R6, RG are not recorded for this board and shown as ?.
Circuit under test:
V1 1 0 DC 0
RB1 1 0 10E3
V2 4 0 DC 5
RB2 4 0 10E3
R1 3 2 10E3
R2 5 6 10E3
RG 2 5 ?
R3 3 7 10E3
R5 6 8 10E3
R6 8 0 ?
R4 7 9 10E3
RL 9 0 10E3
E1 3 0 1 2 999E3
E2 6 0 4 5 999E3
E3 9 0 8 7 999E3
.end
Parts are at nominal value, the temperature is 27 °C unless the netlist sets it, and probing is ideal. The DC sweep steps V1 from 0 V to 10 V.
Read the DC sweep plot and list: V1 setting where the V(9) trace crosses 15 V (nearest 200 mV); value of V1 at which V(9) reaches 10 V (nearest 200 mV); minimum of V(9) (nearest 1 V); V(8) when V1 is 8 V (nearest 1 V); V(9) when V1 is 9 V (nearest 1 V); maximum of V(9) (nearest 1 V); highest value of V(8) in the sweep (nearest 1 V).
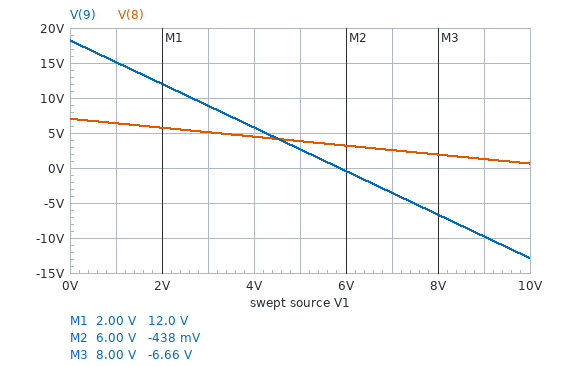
1.0 V
2.6 V
-13 V
2 V
-10 V
18 V
7 V
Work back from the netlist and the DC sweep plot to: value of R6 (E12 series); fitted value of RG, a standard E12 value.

33 kΩ
12 kΩ
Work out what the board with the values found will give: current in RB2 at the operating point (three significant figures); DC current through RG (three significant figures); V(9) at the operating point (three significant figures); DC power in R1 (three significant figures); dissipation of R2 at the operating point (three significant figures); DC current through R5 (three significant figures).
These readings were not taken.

500 µA
417 µA
18.2 V
1.74 mW
1.74 mW
213 µA
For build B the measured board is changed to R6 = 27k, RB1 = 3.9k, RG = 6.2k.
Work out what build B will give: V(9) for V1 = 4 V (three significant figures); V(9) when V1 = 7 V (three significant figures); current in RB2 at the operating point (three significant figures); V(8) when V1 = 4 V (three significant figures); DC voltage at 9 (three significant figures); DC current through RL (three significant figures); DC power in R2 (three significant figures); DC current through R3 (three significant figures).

7.26 V
-7.64 V
500 µA
4.83 V
27.1 V
2.71 mA
6.50 mW
1.76 mA
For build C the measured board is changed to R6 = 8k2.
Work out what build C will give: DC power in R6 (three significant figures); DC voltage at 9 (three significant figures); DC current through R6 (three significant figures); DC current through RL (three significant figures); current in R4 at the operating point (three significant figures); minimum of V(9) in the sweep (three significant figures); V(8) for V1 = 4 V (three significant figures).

2.08 mW
12.4 V
504 µA
1.24 mA
830 µA
-13.4 V
2.63 V
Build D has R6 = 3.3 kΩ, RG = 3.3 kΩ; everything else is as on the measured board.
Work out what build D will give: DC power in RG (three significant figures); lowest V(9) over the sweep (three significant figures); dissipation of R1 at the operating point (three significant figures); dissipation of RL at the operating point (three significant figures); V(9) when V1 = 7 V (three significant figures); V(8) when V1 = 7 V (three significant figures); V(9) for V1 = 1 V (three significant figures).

7.58 mW
-30.2 V
23.0 mW
63.3 mW
-13.6 V
-263 mV
19.6 V
